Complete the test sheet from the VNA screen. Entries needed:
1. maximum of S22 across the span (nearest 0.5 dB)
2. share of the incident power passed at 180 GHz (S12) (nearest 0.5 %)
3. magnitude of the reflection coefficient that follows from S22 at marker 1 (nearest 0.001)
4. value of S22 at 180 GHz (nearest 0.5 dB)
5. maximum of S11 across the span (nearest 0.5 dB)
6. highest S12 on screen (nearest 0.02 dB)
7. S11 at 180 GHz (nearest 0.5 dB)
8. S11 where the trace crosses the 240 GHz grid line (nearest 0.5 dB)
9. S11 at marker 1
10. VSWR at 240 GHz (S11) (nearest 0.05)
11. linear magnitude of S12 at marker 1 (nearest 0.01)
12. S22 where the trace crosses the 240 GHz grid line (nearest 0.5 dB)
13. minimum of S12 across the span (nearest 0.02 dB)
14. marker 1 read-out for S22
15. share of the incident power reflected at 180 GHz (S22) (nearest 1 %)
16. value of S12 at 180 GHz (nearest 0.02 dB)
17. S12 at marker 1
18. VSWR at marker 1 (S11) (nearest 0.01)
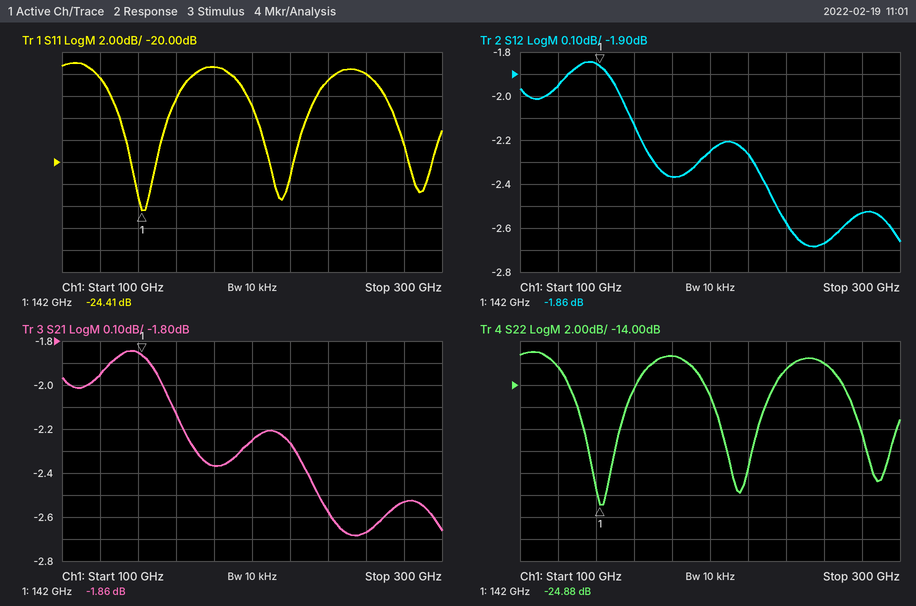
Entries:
-11.0 dB
58.0 %
0.057
-11.5 dB
-11.0 dB
-1.84 dB
-11.5 dB
-12.5 dB
-24.41 dB
1.60
0.81
-12.5 dB
-2.68 dB
-24.88 dB
7 %
-2.36 dB
-1.86 dB
1.13
